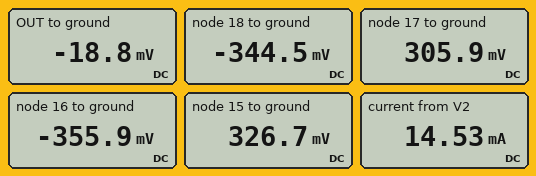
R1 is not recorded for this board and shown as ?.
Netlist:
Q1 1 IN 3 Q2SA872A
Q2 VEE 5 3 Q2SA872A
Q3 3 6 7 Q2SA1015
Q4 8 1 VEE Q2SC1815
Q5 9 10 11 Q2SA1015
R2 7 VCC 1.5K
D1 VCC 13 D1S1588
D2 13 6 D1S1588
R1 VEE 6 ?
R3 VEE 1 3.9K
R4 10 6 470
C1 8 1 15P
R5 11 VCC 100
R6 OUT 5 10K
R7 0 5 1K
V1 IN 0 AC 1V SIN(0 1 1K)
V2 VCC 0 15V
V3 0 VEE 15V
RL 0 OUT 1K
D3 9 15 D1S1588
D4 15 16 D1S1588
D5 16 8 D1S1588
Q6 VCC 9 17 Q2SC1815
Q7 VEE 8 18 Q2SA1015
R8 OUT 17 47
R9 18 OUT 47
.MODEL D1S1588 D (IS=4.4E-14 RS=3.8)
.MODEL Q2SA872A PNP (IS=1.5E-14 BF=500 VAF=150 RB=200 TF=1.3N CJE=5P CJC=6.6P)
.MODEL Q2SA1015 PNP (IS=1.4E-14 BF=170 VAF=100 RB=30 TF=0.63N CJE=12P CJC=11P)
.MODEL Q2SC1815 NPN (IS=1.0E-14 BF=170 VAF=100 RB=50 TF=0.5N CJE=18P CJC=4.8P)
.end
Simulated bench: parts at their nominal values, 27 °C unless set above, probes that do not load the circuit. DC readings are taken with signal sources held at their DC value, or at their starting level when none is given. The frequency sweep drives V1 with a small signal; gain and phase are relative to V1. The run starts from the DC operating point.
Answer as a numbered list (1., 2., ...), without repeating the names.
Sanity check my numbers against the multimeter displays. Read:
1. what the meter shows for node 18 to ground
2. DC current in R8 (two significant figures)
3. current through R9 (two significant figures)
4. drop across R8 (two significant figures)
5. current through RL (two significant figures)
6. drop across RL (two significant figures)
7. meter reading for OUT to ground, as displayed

1. -344.5 mV
2. 6.9 mA
3. 6.9 mA
4. 320 mV
5. 19 µA
6. 19 mV
7. -18.8 mV
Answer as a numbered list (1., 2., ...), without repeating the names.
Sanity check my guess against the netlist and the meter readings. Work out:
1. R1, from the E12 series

1. 18 kΩ
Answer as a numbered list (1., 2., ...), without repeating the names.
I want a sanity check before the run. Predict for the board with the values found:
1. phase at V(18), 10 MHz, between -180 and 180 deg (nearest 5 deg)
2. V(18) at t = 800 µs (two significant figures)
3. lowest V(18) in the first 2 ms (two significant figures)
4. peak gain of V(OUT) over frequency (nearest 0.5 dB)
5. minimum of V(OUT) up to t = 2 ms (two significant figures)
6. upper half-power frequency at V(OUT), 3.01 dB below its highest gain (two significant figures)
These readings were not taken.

1. -125 deg
2. -11 V
3. -12 V
4. 21.0 dB
5. -11 V
6. 4.9 MHz
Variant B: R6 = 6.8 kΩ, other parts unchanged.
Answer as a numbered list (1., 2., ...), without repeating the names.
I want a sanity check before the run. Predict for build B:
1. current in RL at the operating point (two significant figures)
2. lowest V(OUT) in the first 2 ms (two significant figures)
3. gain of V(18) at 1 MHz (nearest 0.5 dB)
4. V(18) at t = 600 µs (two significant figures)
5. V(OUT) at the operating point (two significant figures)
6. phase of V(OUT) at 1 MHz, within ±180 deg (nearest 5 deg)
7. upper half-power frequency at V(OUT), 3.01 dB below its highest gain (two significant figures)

1. 13 µA
2. -7.8 V
3. 18.0 dB
4. -5.0 V
5. -13 mV
6. -10 deg
7. 7.3 MHz
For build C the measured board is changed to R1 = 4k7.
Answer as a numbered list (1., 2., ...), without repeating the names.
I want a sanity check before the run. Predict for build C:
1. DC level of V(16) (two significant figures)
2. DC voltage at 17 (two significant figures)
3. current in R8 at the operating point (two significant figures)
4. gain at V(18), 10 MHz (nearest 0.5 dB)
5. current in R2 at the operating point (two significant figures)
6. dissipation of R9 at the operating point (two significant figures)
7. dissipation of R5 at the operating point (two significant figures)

1. -420 mV
2. 250 mV
3. 7.1 mA
4. 12.0 dB
5. 500 µA
6. 2.4 mW
7. 4.4 mW
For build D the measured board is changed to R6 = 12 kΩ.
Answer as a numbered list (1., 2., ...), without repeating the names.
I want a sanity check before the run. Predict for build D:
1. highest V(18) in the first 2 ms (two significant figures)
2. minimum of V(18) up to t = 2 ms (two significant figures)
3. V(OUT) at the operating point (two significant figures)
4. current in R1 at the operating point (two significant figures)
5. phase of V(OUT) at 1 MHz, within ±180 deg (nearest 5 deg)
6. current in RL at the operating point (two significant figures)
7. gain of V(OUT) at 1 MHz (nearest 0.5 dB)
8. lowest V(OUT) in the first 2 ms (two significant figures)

1. 13 V
2. -14 V
3. -22 mV
4. 1.6 mA
5. -20 deg
6. 22 µA
7. 22.0 dB
8. -13 V
